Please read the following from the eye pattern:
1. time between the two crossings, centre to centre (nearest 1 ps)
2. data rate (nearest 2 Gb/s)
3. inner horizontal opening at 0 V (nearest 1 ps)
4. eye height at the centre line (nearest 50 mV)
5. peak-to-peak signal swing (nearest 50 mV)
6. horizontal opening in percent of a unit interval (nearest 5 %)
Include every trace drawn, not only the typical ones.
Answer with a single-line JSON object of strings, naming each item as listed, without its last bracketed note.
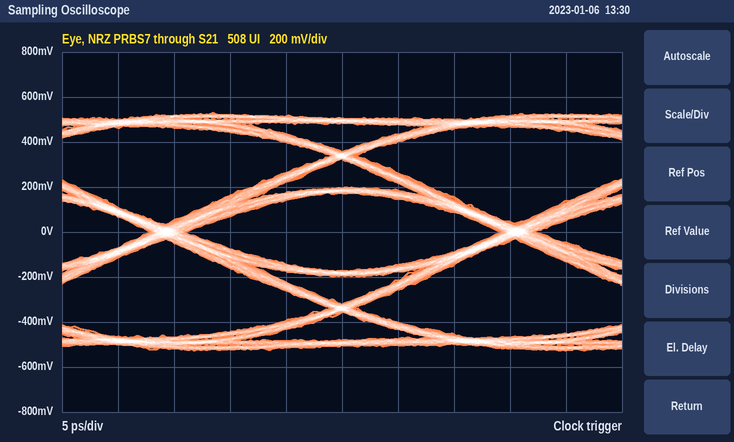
{"time between the two crossings, centre to centre": "31 ps", "data rate": "32 Gb/s", "inner horizontal opening at 0 V": "28 ps", "eye height at the centre line": "350 mV", "peak-to-peak signal swing": "1.05 V", "horizontal opening in percent of a unit interval": "90 %"}
